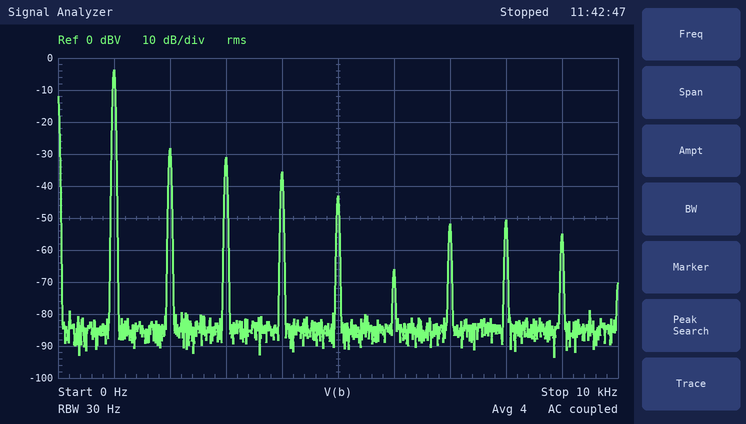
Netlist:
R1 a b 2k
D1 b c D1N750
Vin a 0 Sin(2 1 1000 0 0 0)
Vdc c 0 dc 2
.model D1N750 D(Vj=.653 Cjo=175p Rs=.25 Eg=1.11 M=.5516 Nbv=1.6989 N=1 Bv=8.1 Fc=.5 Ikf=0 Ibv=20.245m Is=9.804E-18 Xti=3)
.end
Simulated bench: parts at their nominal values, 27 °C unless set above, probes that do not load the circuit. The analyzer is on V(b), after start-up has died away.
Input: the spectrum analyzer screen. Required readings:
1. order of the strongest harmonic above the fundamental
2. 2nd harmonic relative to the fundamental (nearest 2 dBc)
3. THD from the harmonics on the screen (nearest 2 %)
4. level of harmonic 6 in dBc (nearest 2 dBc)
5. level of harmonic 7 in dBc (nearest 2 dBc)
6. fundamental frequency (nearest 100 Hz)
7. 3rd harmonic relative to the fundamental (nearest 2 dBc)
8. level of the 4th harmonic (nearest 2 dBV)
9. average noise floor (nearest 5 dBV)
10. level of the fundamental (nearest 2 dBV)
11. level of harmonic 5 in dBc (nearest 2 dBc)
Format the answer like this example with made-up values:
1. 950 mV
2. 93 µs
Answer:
1. 2
2. -24 dBc
3. 8 %
4. -62 dBc
5. -48 dBc
6. 1.0 kHz
7. -28 dBc
8. -36 dBV
9. -85 dBV
10. -4 dBV
11. -40 dBc
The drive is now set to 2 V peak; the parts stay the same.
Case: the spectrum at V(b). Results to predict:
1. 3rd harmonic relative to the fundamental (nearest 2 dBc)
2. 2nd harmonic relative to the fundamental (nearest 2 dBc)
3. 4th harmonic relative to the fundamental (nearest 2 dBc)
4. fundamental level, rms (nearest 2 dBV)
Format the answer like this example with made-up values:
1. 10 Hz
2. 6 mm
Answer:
1. -22 dBc
2. -14 dBc
3. -48 dBc
4. 0 dBV
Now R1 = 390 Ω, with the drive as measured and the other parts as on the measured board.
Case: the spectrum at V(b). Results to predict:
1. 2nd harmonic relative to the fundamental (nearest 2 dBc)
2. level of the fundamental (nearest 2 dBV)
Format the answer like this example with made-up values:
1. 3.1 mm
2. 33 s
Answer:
1. -26 dBc
2. -4 dBV
